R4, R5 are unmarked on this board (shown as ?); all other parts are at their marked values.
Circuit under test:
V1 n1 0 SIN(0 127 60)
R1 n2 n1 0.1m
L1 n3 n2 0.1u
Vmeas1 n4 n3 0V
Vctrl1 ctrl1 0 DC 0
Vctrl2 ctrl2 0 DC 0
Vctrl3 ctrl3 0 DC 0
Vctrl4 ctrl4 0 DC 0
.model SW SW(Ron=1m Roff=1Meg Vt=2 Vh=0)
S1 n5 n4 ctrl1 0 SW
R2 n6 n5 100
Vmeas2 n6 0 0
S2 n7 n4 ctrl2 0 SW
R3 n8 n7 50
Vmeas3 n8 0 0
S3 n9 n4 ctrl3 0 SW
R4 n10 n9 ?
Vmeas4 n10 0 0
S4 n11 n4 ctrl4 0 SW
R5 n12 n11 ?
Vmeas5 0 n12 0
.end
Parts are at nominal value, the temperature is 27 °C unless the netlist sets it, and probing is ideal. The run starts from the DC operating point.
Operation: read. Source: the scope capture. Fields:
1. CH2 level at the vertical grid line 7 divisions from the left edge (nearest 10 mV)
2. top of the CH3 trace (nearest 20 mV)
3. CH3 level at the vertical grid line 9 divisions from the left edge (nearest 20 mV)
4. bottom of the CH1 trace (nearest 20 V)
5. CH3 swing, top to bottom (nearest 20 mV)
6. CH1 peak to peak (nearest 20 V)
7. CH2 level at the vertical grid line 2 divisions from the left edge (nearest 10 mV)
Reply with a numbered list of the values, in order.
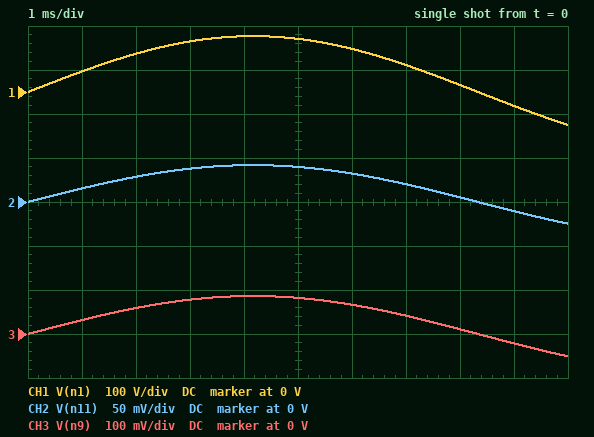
1. 20 mV
2. 80 mV
3. -20 mV
4. -80 V
5. 140 mV
6. 200 V
7. 30 mV
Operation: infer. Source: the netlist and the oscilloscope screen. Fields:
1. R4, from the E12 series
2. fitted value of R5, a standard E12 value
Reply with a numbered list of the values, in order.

1. 680 Ω
2. 330 Ω
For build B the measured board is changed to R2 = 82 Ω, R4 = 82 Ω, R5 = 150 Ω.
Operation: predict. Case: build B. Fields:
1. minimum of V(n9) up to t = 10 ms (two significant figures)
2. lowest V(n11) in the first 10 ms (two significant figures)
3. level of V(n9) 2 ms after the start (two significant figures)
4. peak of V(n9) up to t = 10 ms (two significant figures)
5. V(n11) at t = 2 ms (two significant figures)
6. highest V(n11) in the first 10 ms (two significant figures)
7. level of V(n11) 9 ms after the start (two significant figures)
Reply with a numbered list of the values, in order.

1. -6.1 mV
2. -11 mV
3. 7.1 mV
4. 10 mV
5. 13 mV
6. 19 mV
7. -4.7 mV
